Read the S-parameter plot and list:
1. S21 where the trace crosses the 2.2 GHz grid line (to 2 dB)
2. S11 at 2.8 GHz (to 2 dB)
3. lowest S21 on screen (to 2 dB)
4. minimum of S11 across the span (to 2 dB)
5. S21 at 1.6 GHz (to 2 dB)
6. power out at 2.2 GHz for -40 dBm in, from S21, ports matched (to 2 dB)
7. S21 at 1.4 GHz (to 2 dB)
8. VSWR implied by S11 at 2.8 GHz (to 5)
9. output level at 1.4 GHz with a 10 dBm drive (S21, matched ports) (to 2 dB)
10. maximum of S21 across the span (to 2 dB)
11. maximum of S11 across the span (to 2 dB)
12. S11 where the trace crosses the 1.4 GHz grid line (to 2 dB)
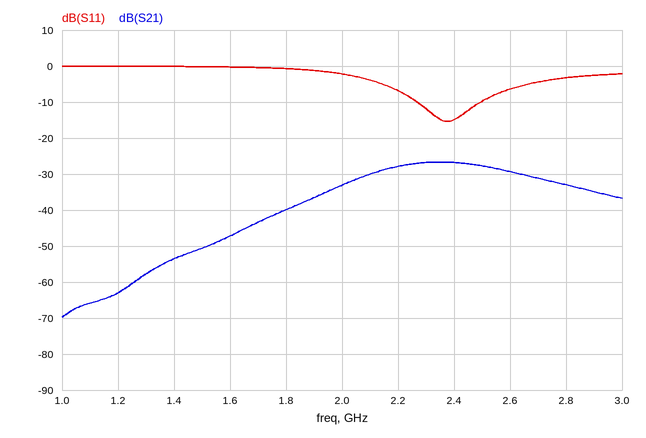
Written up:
-28 dB
-4 dB
-70 dB
-16 dB
-48 dB
-68 dBm
-54 dB
5
-44 dBm
-26 dB
0 dB
0 dB
